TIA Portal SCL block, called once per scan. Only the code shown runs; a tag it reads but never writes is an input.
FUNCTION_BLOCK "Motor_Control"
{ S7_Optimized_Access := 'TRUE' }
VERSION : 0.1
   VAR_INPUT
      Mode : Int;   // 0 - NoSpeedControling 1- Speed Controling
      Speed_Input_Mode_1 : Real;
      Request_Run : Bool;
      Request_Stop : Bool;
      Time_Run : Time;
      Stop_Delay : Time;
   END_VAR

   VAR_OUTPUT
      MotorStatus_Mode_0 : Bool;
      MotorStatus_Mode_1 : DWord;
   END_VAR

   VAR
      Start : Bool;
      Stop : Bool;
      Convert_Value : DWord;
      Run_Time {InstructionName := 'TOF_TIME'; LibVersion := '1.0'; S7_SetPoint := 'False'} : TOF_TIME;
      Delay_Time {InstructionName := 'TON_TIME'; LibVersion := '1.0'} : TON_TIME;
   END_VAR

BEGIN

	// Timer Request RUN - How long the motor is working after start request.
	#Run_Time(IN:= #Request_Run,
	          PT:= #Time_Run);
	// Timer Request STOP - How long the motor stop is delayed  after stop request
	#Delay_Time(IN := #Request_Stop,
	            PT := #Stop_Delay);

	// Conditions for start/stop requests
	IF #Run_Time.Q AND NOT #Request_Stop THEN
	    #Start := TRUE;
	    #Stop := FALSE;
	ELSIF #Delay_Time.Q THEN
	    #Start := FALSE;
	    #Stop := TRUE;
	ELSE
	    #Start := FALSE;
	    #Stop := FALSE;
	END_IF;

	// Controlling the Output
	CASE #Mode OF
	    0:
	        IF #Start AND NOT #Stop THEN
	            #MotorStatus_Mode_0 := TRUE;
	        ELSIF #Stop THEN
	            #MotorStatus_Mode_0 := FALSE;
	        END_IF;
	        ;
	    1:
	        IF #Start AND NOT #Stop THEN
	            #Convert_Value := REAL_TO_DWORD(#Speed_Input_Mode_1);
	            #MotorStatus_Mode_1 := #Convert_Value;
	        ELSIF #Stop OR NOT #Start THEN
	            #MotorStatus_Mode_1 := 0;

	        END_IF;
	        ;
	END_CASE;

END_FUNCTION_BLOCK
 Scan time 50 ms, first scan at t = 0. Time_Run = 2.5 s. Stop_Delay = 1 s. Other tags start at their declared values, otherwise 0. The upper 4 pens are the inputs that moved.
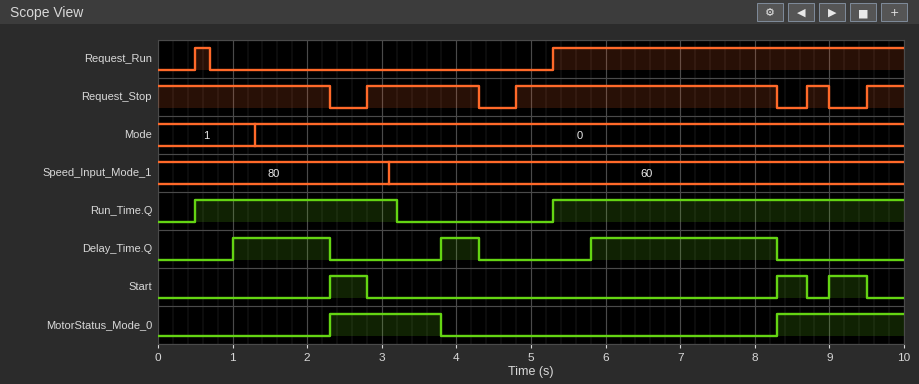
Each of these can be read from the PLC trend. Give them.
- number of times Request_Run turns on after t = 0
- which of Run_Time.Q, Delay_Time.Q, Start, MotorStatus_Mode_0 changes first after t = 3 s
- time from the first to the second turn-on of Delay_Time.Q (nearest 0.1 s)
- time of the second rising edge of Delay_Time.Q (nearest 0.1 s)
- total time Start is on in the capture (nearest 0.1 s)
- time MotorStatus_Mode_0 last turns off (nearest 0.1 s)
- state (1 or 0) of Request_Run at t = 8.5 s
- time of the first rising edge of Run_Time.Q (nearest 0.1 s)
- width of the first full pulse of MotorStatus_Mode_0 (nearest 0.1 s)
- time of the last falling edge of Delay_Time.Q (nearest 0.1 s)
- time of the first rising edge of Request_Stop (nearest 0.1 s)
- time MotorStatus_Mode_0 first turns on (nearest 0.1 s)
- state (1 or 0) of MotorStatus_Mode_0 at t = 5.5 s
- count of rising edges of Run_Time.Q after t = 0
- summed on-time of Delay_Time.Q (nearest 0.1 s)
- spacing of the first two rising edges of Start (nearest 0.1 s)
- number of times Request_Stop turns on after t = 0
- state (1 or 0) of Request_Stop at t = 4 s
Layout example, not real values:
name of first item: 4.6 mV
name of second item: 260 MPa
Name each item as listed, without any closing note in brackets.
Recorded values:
number of times Request_Run turns on after t = 0: 2
which of Run_Time.Q, Delay_Time.Q, Start, MotorStatus_Mode_0 changes first after t = 3 s: Run_Time.Q
time from the first to the second turn-on of Delay_Time.Q: 2.8 s
time of the second rising edge of Delay_Time.Q: 3.8 s
total time Start is on in the capture: 1.4 s
time MotorStatus_Mode_0 last turns off: 3.8 s
state (1 or 0) of Request_Run at t = 8.5 s: 1
time of the first rising edge of Run_Time.Q: 0.5 s
width of the first full pulse of MotorStatus_Mode_0: 1.5 s
time of the last falling edge of Delay_Time.Q: 8.3 s
time of the first rising edge of Request_Stop: 2.8 s
time MotorStatus_Mode_0 first turns on: 2.3 s
state (1 or 0) of MotorStatus_Mode_0 at t = 5.5 s: 0
count of rising edges of Run_Time.Q after t = 0: 2
summed on-time of Delay_Time.Q: 4.3 s
spacing of the first two rising edges of Start: 6.0 s
number of times Request_Stop turns on after t = 0: 4
state (1 or 0) of Request_Stop at t = 4 s: 1
